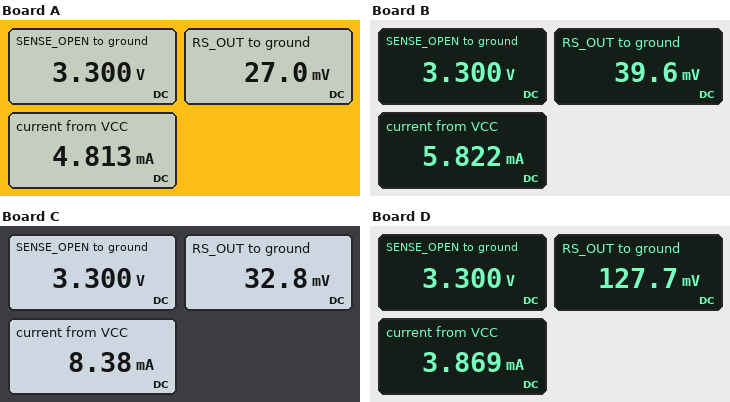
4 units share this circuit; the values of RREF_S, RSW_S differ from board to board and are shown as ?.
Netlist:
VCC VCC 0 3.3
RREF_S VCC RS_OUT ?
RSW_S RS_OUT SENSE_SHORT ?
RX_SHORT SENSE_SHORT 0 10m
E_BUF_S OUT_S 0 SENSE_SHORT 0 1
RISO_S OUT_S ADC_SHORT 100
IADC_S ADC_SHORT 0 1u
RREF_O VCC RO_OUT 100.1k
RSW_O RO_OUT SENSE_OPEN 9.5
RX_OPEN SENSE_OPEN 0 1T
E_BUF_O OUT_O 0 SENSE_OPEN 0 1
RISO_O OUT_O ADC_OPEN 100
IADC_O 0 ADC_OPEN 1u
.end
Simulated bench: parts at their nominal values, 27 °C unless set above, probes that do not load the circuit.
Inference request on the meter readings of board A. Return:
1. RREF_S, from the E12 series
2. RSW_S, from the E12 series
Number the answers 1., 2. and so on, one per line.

1. 680 Ω
2. 5.6 Ω
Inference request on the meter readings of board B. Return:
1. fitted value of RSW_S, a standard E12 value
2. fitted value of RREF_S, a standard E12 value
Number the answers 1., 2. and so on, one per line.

1. 6.8 Ω
2. 560 Ω
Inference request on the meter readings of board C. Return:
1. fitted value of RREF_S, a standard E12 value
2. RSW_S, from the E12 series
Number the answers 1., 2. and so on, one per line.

1. 390 Ω
2. 3.9 Ω
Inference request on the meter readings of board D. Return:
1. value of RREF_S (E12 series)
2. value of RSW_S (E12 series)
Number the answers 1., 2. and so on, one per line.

1. 820 Ω
2. 33 Ω
